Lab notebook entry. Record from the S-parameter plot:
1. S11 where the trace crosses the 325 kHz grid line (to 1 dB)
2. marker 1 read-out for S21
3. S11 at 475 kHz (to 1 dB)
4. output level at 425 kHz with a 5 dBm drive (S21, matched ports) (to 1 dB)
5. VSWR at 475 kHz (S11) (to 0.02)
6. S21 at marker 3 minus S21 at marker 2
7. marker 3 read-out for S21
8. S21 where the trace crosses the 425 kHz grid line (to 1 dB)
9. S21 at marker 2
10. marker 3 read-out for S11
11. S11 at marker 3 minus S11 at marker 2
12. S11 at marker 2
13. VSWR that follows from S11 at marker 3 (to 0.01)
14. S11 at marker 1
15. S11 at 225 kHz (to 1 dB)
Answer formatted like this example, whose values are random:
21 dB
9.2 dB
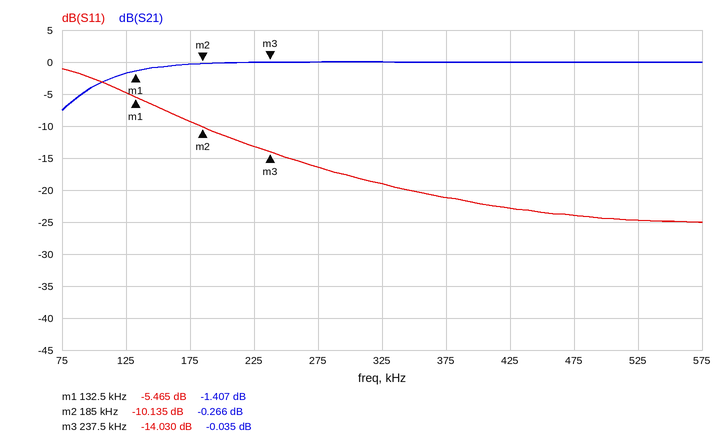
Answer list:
-19 dB
-1.407 dB
-24 dB
5 dBm
1.14
0.231 dB
-0.035 dB
0 dB
-0.266 dB
-14.030 dB
-3.895 dB
-10.135 dB
1.50
-5.465 dB
-13 dB
